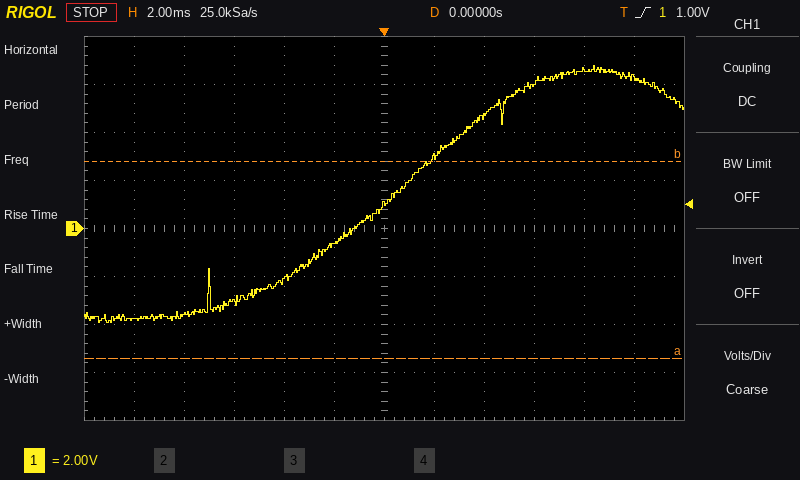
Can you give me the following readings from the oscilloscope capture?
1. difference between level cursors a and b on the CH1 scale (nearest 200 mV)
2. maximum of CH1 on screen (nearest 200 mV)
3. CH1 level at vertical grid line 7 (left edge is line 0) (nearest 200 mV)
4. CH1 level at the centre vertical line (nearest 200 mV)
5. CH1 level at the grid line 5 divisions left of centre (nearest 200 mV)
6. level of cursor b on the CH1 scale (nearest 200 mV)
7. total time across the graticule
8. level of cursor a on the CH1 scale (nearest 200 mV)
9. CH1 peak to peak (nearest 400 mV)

8.2 V
6.8 V
3.0 V
1.0 V
-3.8 V
2.8 V
24 ms
-5.4 V
10.8 V
